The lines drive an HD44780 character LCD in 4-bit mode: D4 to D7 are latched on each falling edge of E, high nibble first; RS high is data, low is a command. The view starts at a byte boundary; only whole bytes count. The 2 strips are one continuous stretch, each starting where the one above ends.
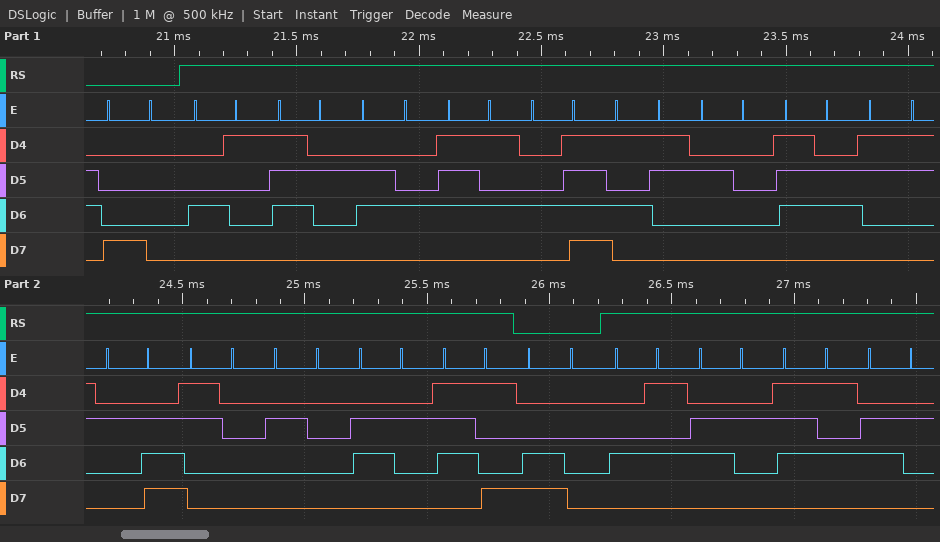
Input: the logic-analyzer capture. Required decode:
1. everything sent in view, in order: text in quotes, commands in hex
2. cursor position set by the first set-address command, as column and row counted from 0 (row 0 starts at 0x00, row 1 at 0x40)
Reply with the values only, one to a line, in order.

0x80 "ArduOS v3.0 by" 0xC0 "Ebub"
column 0, row 0
